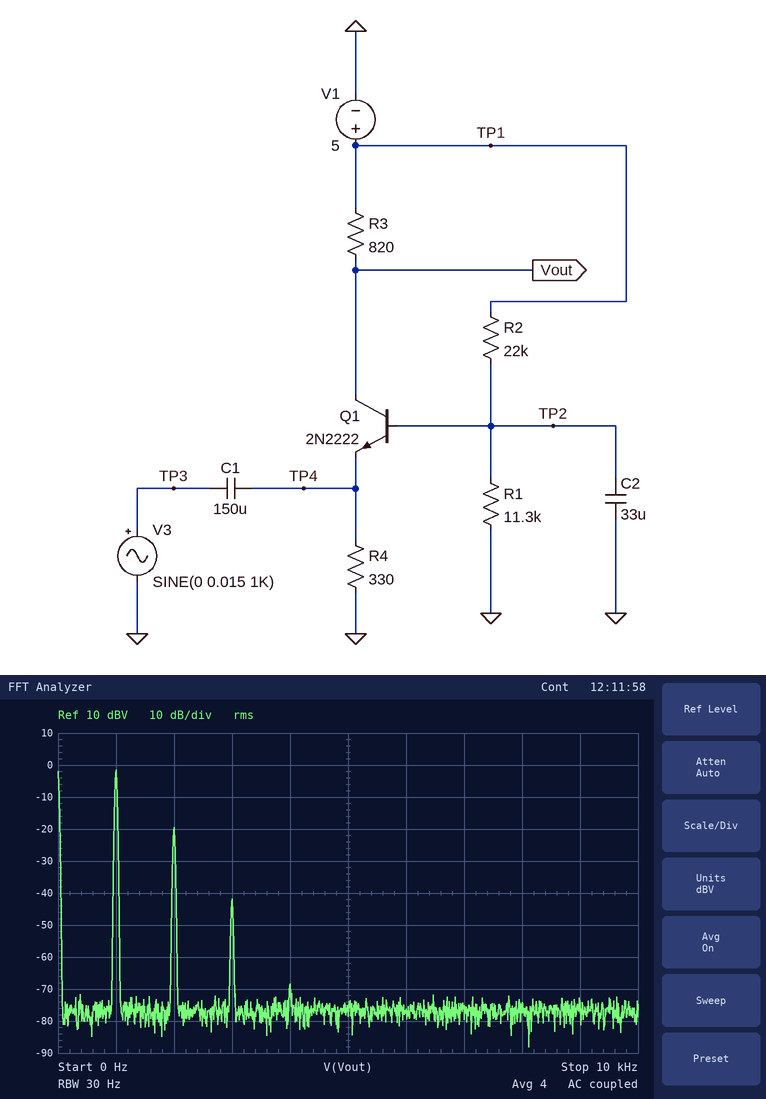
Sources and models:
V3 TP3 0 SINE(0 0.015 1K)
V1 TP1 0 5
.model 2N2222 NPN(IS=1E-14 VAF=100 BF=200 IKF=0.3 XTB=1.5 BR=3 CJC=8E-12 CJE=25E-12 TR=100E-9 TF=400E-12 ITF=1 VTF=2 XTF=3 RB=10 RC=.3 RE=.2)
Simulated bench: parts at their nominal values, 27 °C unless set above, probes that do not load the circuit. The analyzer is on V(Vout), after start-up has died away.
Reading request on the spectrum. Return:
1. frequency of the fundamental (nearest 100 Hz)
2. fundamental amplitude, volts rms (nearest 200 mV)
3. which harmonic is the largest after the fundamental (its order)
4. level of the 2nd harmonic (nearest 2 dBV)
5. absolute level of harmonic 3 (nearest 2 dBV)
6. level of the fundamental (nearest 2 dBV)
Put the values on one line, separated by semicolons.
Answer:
1.0 kHz; 800 mV; 2; -20 dBV; -42 dBV; -2 dBV
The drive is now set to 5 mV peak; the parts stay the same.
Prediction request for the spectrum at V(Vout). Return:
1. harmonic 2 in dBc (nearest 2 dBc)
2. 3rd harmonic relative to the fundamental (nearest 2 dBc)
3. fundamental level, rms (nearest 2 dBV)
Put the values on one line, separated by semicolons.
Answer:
-28 dBc; -60 dBc; -10 dBV
